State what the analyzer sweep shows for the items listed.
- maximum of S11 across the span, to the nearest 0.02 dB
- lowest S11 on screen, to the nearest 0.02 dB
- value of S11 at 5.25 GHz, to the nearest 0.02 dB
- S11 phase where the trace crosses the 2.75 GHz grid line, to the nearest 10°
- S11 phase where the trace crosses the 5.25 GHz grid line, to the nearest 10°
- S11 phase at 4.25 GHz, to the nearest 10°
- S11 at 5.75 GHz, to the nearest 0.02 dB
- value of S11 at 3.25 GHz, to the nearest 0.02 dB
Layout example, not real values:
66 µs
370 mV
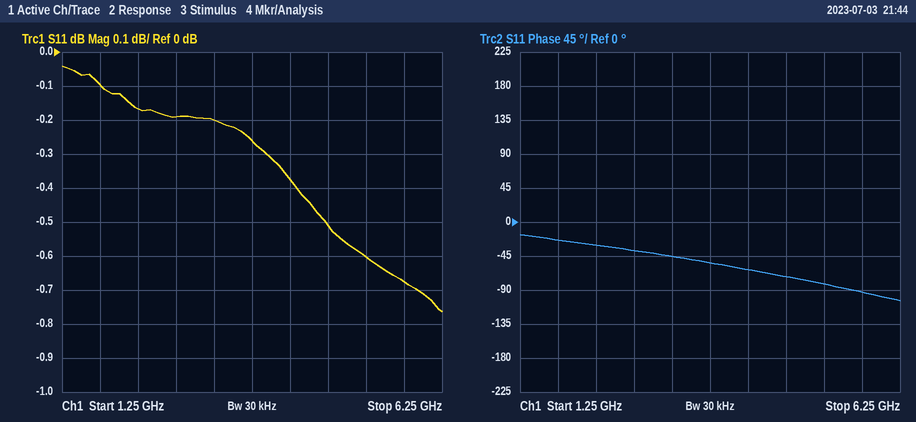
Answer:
-0.04 dB
-0.76 dB
-0.60 dB
-40°
-80°
-60°
-0.68 dB
-0.20 dB
